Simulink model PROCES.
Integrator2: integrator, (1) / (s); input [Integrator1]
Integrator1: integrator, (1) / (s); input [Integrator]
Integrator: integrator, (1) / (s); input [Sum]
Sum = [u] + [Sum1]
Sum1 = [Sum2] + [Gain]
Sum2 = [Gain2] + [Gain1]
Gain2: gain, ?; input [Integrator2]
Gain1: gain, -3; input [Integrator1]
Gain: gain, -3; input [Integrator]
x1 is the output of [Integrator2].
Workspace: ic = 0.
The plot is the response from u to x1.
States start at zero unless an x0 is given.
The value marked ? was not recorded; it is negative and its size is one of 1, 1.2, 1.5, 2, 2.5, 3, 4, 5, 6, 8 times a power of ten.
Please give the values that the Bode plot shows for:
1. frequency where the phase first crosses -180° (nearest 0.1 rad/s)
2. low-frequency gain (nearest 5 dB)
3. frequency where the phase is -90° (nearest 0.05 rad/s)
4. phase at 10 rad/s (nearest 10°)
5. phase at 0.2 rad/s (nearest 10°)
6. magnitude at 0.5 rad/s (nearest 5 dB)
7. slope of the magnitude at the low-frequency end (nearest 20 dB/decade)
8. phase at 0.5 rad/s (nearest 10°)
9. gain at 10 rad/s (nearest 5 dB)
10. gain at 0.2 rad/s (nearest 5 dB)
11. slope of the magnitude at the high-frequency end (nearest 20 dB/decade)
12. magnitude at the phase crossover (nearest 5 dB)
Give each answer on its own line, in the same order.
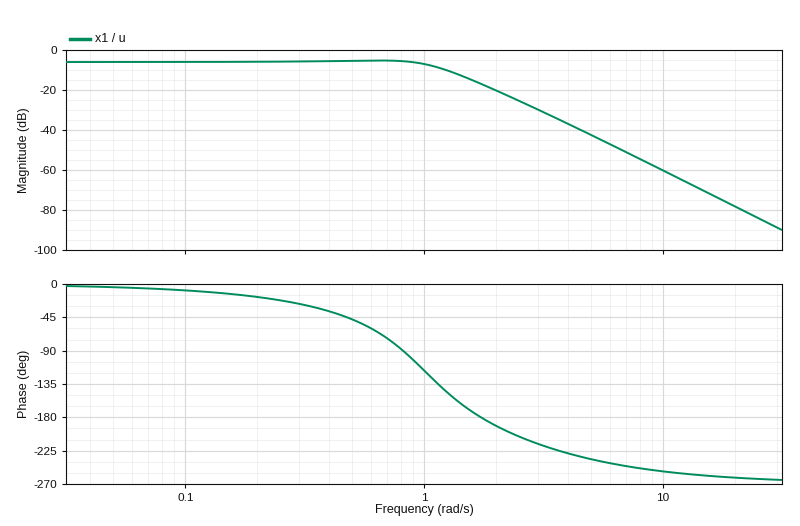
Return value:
1.7 rad/s
-5 dB
0.80 rad/s
-250°
-20°
-5 dB
0 dB/decade
-50°
-60 dB
-5 dB
-60 dB/decade
-15 dB
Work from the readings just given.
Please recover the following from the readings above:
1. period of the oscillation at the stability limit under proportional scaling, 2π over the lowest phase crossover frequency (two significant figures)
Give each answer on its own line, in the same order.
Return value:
3.7 s
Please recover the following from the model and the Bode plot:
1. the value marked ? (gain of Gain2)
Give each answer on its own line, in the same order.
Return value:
-2
